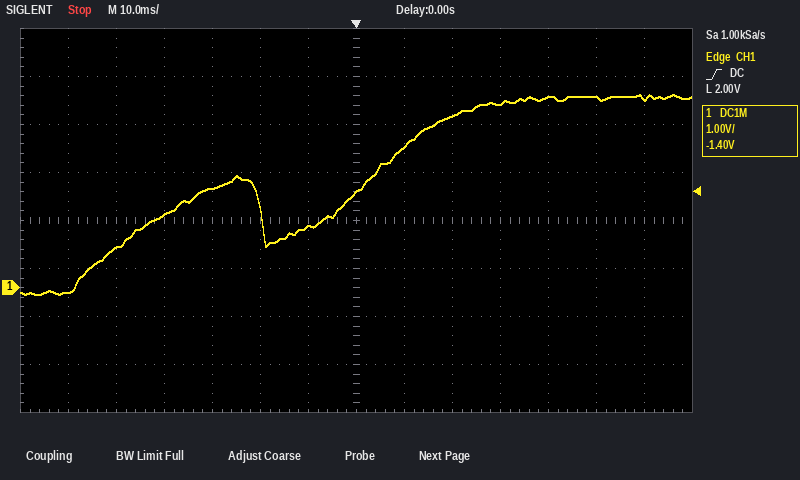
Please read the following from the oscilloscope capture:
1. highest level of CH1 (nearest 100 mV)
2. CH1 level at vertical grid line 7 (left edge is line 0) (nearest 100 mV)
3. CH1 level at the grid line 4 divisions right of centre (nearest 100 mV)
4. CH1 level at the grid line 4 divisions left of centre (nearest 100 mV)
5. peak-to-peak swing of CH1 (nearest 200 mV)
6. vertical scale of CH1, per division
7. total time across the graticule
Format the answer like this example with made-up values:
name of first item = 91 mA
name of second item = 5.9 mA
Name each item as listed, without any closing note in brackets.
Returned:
highest level of CH1 = 4.0 V
CH1 level at vertical grid line 7 (left edge is line 0) = 2.0 V
CH1 level at the grid line 4 divisions right of centre = 4.0 V
CH1 level at the grid line 4 divisions left of centre = 1.5 V
peak-to-peak swing of CH1 = 4.2 V
vertical scale of CH1, per division = 1 V
total time across the graticule = 140 ms
